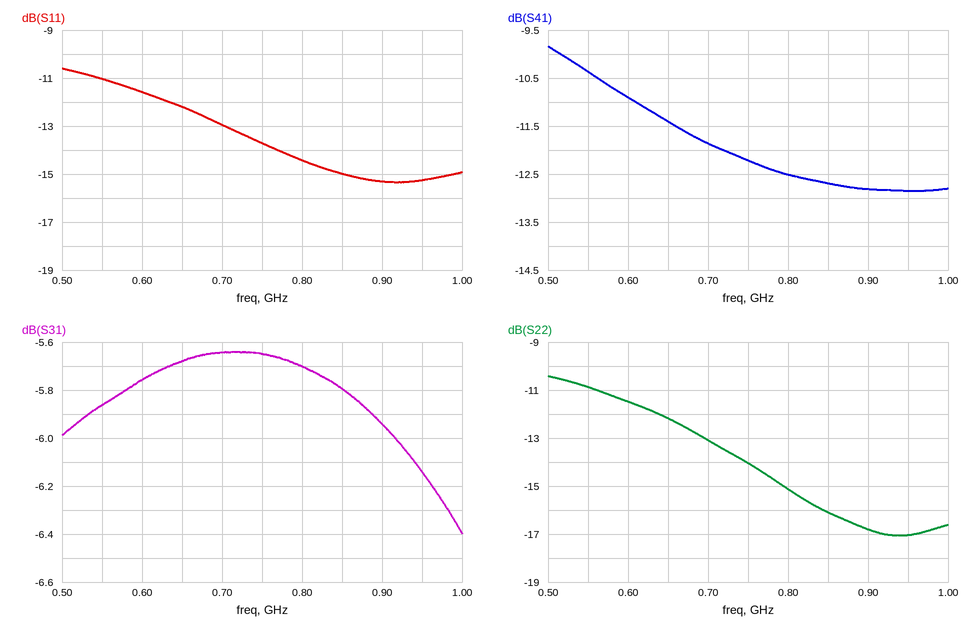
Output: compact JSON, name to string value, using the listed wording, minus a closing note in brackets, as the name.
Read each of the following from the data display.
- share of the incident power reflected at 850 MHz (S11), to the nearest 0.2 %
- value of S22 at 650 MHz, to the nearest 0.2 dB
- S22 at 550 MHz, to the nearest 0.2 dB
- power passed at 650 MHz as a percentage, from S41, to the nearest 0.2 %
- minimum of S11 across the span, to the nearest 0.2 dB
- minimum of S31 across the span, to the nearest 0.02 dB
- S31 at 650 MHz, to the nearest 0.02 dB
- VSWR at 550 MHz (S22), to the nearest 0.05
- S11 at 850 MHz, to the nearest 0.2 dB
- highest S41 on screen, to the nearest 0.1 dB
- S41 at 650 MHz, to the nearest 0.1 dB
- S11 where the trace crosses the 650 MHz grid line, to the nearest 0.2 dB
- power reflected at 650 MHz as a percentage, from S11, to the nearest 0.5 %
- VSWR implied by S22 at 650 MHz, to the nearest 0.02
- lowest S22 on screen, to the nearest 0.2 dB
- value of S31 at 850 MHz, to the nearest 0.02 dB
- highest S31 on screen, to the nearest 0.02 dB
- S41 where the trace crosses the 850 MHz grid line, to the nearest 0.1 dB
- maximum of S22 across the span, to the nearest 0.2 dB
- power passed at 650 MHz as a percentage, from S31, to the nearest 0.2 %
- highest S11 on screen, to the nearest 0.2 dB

{"share of the incident power reflected at 850 MHz (S11), to the nearest 0.2 %": "3.2 %", "value of S22 at 650 MHz, to the nearest 0.2 dB": "-12.2 dB", "S22 at 550 MHz, to the nearest 0.2 dB": "-10.8 dB", "power passed at 650 MHz as a percentage, from S41, to the nearest 0.2 %": "7.2 %", "minimum of S11 across the span, to the nearest 0.2 dB": "-15.4 dB", "minimum of S31 across the span, to the nearest 0.02 dB": "-6.40 dB", "S31 at 650 MHz, to the nearest 0.02 dB": "-5.68 dB", "VSWR at 550 MHz (S22), to the nearest 0.05": "1.80", "S11 at 850 MHz, to the nearest 0.2 dB": "-15.0 dB", "highest S41 on screen, to the nearest 0.1 dB": "-9.8 dB", "S41 at 650 MHz, to the nearest 0.1 dB": "-11.4 dB", "S11 where the trace crosses the 650 MHz grid line, to the nearest 0.2 dB": "-12.2 dB", "power reflected at 650 MHz as a percentage, from S11, to the nearest 0.5 %": "6.0 %", "VSWR implied by S22 at 650 MHz, to the nearest 0.02": "1.66", "lowest S22 on screen, to the nearest 0.2 dB": "-17.0 dB", "value of S31 at 850 MHz, to the nearest 0.02 dB": "-5.80 dB", "highest S31 on screen, to the nearest 0.02 dB": "-5.64 dB", "S41 where the trace crosses the 850 MHz grid line, to the nearest 0.1 dB": "-12.7 dB", "maximum of S22 across the span, to the nearest 0.2 dB": "-10.4 dB", "power passed at 650 MHz as a percentage, from S31, to the nearest 0.2 %": "27.0 %", "highest S11 on screen, to the nearest 0.2 dB": "-10.6 dB"}
